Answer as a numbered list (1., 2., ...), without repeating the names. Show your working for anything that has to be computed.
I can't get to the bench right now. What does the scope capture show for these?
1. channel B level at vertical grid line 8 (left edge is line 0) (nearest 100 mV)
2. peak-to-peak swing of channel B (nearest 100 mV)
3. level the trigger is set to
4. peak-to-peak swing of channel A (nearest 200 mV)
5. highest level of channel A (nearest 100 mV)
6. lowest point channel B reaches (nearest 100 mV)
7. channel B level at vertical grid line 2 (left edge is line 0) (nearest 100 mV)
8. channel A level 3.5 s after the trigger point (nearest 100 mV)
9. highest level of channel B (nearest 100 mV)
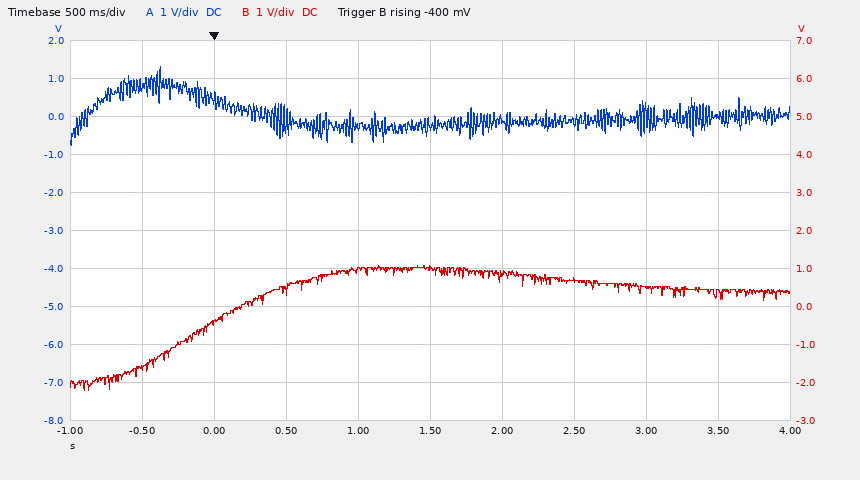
1. 500 mV
2. 1.1 V − (-2.2 V) = 3.3 V
3. -400 mV
4. 2.0 V
5. 1.3 V
6. -2.2 V
7. -400 mV
8. 0.0 V
9. 1.1 V
